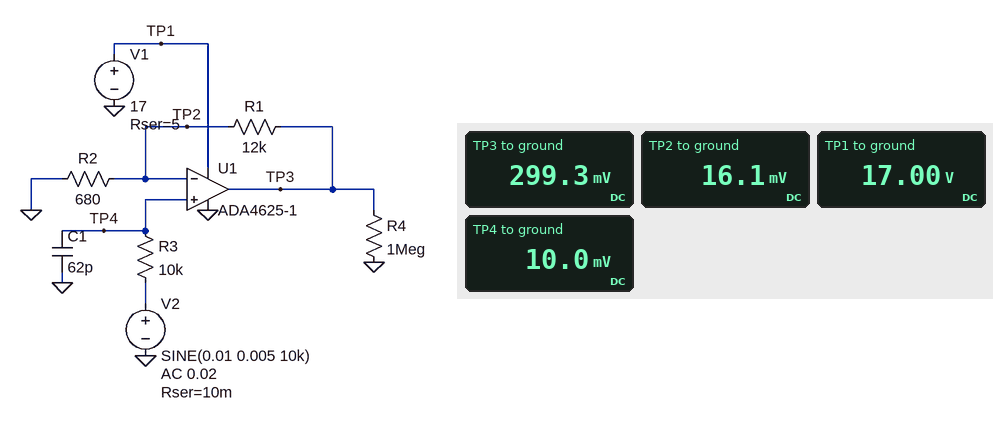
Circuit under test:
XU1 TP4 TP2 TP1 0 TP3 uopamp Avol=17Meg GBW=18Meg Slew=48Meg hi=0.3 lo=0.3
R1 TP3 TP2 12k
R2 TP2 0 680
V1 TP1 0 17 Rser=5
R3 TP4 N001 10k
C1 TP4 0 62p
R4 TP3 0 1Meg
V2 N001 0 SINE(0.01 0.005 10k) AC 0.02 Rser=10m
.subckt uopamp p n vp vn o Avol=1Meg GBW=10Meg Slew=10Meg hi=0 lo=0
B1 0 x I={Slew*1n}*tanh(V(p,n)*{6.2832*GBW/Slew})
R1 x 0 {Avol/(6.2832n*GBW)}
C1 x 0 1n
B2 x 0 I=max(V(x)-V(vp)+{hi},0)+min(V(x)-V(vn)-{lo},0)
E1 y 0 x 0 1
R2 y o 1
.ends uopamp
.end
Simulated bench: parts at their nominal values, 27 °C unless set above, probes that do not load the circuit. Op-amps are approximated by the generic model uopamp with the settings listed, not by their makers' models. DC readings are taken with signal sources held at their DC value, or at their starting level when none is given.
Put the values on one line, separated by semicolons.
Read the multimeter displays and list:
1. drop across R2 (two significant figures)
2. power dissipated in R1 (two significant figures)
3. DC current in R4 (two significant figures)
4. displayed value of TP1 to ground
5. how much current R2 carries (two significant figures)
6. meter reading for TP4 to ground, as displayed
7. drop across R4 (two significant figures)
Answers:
16 mV; 6.7 µW; 300 nA; 17.00 V; 24 µA; 10.0 mV; 300 mV
